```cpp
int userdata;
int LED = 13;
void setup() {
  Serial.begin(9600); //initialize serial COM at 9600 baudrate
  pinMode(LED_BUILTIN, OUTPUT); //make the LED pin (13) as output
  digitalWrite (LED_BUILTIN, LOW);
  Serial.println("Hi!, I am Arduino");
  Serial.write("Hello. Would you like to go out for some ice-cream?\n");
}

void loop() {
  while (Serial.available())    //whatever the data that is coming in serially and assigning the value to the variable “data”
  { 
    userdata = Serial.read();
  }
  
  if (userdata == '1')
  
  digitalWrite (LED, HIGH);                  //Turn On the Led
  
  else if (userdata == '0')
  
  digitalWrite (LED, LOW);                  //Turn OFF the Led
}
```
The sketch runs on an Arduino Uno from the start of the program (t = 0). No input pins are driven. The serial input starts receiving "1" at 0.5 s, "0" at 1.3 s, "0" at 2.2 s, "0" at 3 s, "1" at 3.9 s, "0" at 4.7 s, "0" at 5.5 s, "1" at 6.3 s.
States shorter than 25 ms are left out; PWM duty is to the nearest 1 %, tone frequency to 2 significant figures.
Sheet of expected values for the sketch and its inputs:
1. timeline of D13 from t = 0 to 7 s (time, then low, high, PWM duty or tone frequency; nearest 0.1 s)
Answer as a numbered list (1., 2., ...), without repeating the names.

1. 0 s low; 0.5 s high; 1.3 s low; 3.9 s high; 4.7 s low; 6.3 s high
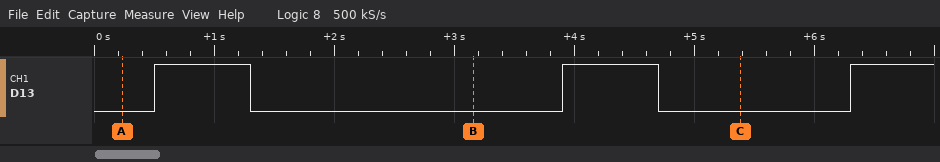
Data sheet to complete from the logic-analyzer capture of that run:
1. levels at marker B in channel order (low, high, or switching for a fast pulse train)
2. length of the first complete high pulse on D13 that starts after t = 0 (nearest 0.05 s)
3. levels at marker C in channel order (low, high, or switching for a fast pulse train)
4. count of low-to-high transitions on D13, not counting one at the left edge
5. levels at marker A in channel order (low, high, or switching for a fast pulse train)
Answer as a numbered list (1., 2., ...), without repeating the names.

1. D13 low
2. 0.80 s
3. D13 low
4. 3
5. D13 low
